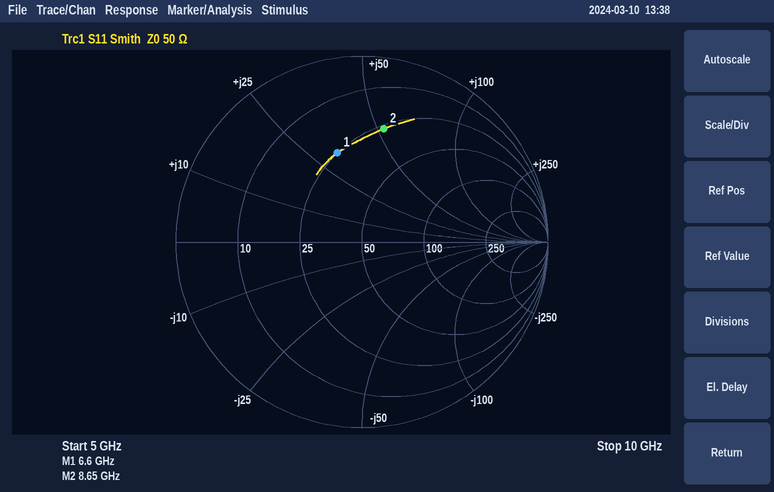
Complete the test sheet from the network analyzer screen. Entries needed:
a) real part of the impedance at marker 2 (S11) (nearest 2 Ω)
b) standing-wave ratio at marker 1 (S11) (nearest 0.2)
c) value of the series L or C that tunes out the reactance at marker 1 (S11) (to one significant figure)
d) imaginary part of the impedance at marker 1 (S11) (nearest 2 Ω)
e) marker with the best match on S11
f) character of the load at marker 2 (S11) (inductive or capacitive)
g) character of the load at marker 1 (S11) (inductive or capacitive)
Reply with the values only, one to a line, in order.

26 Ω
3.0
800 fF
+32 Ω
marker 1
inductive
inductive
